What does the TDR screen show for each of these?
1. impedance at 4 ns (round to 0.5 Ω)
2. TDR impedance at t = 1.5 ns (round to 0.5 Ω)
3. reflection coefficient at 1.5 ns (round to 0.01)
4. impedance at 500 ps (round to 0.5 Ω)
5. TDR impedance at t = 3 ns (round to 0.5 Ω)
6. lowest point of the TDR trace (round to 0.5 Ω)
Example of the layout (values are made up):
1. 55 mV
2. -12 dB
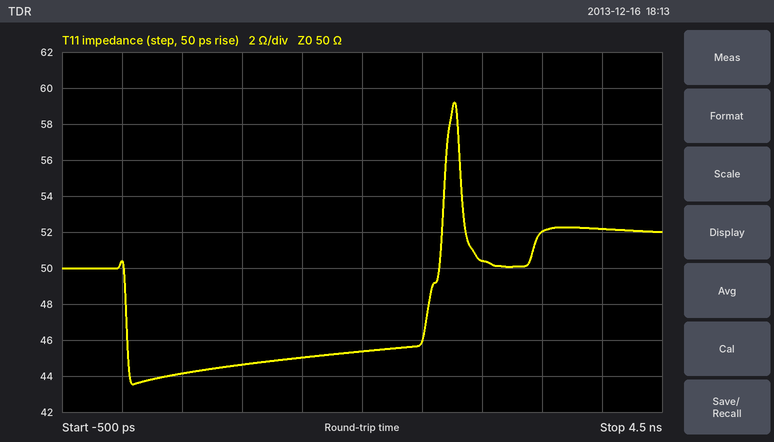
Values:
1. 52.0 Ω
2. 45.0 Ω
3. -0.05
4. 44.0 Ω
5. 50.5 Ω
6. 43.5 Ω
